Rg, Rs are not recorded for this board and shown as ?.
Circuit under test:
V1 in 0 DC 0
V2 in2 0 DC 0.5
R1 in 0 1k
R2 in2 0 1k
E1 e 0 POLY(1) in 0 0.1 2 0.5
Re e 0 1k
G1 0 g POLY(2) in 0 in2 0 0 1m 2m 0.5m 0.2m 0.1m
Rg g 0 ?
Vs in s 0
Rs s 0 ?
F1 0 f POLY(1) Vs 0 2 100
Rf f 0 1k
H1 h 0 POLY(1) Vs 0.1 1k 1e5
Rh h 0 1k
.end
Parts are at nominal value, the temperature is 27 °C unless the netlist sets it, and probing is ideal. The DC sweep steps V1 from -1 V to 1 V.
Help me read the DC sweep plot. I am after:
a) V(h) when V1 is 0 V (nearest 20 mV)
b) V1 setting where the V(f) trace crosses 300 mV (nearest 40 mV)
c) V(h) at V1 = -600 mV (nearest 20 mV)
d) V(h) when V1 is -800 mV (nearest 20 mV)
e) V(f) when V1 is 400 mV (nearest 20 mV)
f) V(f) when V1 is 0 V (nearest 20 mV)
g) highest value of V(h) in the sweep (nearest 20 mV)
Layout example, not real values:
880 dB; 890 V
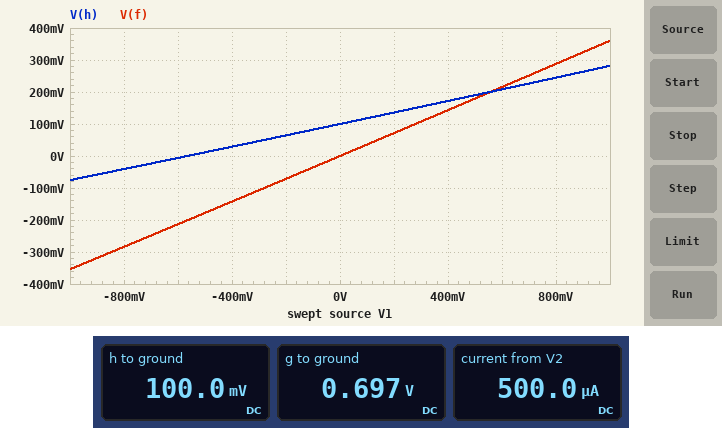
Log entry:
100 mV; 840 mV; 0 V; -40 mV; 140 mV; 0 V; 280 mV
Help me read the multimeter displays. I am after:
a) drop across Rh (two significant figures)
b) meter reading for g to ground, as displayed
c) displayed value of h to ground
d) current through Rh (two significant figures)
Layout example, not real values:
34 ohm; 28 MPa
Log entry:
100 mV; 0.697 V; 100.0 mV; 100 µA
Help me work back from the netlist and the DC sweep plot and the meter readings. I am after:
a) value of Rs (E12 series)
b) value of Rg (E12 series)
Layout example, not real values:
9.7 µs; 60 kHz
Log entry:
5.6 kΩ; 680 Ω
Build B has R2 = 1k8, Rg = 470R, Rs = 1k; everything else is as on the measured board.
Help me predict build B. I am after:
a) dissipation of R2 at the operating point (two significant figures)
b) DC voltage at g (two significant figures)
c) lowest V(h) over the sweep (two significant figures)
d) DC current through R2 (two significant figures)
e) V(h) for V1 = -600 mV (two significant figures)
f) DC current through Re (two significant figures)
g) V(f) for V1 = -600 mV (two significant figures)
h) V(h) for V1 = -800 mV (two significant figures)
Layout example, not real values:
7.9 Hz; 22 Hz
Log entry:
140 µW; 480 mV; -800 mV; 280 µA; -460 mV; 100 µA; -1.2 V; -640 mV
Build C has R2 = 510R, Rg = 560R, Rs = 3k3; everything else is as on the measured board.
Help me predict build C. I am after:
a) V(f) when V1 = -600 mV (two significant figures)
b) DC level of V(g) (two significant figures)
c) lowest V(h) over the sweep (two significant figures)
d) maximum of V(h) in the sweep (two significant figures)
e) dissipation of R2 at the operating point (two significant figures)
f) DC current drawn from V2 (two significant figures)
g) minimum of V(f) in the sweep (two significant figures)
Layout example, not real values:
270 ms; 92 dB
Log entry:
-360 mV; 570 mV; -190 mV; 410 mV; 490 µW; 980 µA; -600 mV
